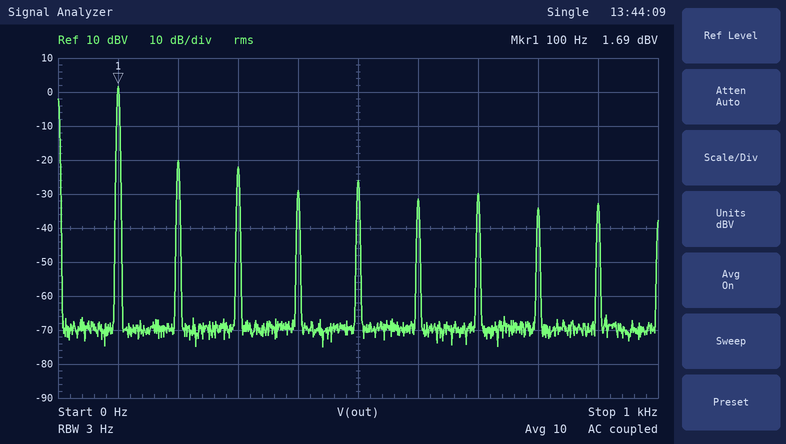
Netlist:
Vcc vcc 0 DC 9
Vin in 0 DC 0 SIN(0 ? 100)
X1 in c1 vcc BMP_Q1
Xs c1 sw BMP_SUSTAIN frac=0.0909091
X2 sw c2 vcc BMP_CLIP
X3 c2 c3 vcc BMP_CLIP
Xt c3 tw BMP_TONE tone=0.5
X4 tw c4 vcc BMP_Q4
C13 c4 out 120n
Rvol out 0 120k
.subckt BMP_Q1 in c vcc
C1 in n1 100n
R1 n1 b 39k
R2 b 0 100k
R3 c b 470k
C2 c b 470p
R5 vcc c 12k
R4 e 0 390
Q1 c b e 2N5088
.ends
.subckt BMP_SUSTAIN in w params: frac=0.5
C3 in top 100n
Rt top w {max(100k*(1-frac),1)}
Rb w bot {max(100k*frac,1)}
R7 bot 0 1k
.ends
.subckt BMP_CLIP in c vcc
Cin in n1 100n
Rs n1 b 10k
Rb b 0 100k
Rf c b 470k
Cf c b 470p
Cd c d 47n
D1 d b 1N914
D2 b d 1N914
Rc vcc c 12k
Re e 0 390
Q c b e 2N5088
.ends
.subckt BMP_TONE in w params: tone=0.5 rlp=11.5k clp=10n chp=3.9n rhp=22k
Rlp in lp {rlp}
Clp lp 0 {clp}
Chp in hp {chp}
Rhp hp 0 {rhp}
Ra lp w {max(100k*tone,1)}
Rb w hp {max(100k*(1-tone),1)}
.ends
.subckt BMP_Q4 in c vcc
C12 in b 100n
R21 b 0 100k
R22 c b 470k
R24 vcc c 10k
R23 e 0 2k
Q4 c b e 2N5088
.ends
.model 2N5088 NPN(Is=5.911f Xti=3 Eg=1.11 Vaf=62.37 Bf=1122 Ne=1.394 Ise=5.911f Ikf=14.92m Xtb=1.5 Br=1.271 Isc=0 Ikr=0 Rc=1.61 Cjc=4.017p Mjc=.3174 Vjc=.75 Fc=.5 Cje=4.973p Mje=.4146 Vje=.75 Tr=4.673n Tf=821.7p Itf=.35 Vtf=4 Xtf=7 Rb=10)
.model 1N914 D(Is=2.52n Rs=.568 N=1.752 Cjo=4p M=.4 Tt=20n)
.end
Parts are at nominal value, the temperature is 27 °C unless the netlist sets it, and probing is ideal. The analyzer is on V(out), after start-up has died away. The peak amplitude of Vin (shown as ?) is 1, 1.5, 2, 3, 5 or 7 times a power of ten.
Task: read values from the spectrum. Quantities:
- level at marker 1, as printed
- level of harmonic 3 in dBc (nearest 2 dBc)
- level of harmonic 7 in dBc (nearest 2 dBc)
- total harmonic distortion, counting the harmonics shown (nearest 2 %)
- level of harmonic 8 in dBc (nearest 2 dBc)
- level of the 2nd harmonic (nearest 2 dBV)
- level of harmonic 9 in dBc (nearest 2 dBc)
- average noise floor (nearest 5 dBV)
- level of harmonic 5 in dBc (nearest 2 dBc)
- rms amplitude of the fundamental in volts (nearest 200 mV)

1.69 dBV
-24 dBc
-32 dBc
12 %
-36 dBc
-20 dBV
-34 dBc
-70 dBV
-28 dBc
1.2 V
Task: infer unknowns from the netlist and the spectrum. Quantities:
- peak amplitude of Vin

2 V
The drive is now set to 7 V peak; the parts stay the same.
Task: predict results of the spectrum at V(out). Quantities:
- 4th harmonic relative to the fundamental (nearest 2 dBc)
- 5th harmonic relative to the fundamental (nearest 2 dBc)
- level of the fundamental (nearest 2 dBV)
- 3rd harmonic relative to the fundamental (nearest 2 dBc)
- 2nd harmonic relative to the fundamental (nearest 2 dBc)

-24 dBc
-30 dBc
2 dBV
-28 dBc
-16 dBc
